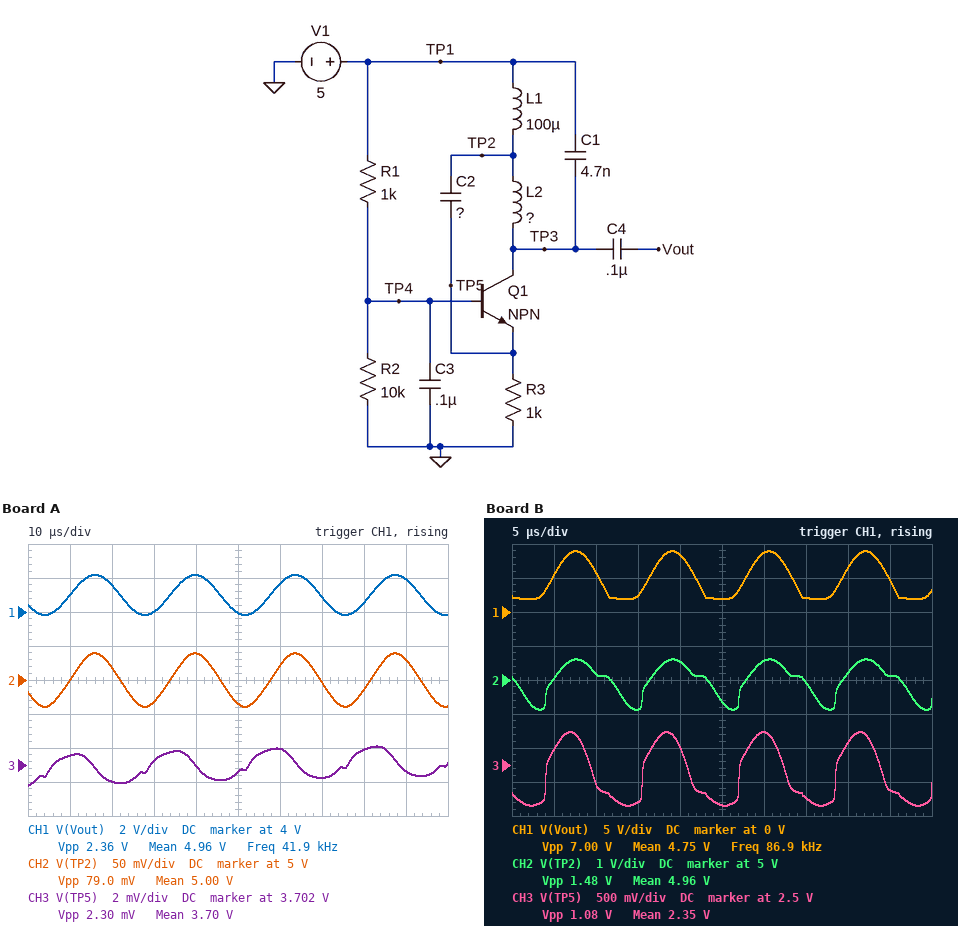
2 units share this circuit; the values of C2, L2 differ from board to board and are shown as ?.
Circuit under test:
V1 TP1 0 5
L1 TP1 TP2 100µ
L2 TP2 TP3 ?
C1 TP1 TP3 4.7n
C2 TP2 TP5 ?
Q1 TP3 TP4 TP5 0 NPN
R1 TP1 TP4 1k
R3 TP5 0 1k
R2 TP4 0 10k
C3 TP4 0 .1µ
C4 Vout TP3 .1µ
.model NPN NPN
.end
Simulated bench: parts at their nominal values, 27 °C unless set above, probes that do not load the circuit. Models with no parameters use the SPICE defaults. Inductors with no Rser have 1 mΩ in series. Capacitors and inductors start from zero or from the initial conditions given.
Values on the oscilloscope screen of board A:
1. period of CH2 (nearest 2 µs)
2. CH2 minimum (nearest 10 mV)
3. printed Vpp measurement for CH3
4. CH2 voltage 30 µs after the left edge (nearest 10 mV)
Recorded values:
24 µs
4.96 V
2.30 mV
4.97 V
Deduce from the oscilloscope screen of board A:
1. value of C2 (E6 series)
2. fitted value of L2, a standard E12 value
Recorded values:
15 nF
3.3 mH
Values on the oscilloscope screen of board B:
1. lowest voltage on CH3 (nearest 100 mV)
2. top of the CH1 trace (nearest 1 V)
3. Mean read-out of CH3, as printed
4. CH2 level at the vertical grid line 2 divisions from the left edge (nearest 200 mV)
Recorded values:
1.9 V
9 V
2.35 V
5.2 V
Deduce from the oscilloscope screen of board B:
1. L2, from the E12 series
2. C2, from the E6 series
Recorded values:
560 µH
22 nF
